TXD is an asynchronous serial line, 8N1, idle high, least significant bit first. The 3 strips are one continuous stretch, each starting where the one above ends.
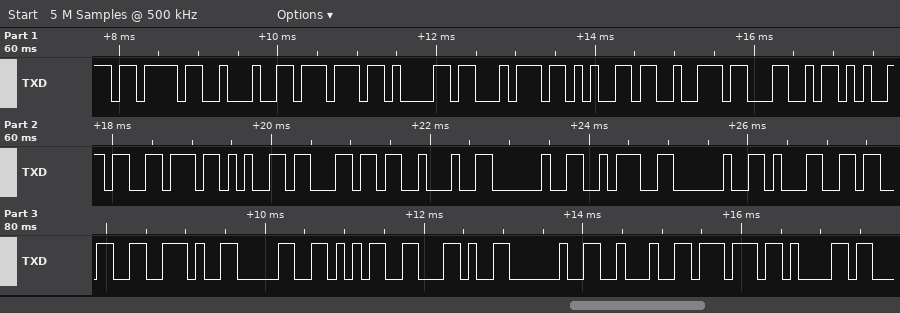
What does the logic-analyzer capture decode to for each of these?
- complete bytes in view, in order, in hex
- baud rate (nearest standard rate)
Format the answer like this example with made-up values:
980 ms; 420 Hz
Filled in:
0x7B 0x22 0x77 0x61 0x74 0x65 0x72 0x4C 0x65 0x76 0x65 0x6C 0x22 0x20 0x3A 0x20 0x31 0x33 0x2E 0x30 0x35 0x2C 0x20 0x22 0x77 0x61; 9600 baud
